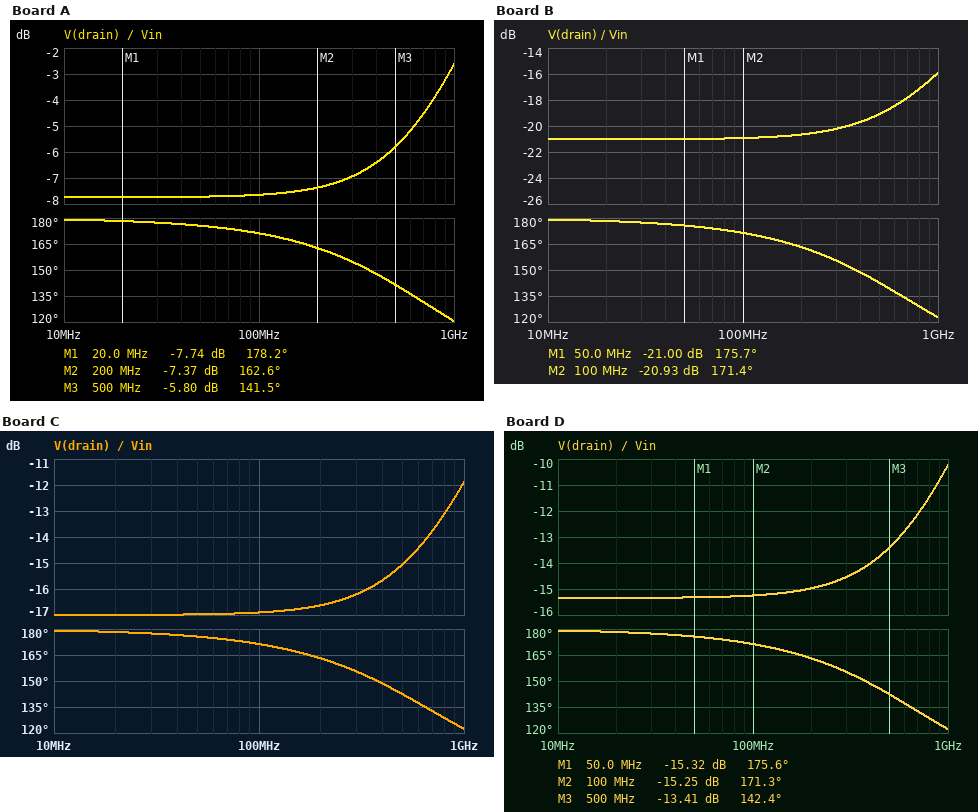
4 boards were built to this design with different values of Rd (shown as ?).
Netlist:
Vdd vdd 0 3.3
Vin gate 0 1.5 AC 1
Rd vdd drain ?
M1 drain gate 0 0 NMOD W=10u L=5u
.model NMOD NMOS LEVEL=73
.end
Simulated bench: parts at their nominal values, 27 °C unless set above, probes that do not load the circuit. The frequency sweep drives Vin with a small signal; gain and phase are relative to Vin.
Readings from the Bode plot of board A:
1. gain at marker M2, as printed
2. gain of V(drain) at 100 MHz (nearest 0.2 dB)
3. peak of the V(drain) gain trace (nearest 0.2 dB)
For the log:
-7.37 dB
-7.6 dB
-2.6 dB
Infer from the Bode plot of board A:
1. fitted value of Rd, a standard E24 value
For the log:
1.8 kΩ
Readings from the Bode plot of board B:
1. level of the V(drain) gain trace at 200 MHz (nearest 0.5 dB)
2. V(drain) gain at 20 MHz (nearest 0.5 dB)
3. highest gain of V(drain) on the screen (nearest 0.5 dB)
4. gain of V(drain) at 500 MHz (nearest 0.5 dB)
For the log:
-20.5 dB
-21.0 dB
-16.0 dB
-19.0 dB
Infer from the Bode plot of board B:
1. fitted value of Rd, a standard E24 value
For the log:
390 Ω
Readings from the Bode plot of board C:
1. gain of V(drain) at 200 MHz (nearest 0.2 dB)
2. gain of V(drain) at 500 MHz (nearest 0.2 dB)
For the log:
-16.6 dB
-15.0 dB
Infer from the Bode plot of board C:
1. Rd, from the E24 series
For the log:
620 Ω
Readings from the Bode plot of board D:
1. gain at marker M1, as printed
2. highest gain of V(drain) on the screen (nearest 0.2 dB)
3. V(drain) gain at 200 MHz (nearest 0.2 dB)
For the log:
-15.32 dB
-10.2 dB
-15.0 dB
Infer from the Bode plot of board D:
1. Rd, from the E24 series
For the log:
750 Ω
